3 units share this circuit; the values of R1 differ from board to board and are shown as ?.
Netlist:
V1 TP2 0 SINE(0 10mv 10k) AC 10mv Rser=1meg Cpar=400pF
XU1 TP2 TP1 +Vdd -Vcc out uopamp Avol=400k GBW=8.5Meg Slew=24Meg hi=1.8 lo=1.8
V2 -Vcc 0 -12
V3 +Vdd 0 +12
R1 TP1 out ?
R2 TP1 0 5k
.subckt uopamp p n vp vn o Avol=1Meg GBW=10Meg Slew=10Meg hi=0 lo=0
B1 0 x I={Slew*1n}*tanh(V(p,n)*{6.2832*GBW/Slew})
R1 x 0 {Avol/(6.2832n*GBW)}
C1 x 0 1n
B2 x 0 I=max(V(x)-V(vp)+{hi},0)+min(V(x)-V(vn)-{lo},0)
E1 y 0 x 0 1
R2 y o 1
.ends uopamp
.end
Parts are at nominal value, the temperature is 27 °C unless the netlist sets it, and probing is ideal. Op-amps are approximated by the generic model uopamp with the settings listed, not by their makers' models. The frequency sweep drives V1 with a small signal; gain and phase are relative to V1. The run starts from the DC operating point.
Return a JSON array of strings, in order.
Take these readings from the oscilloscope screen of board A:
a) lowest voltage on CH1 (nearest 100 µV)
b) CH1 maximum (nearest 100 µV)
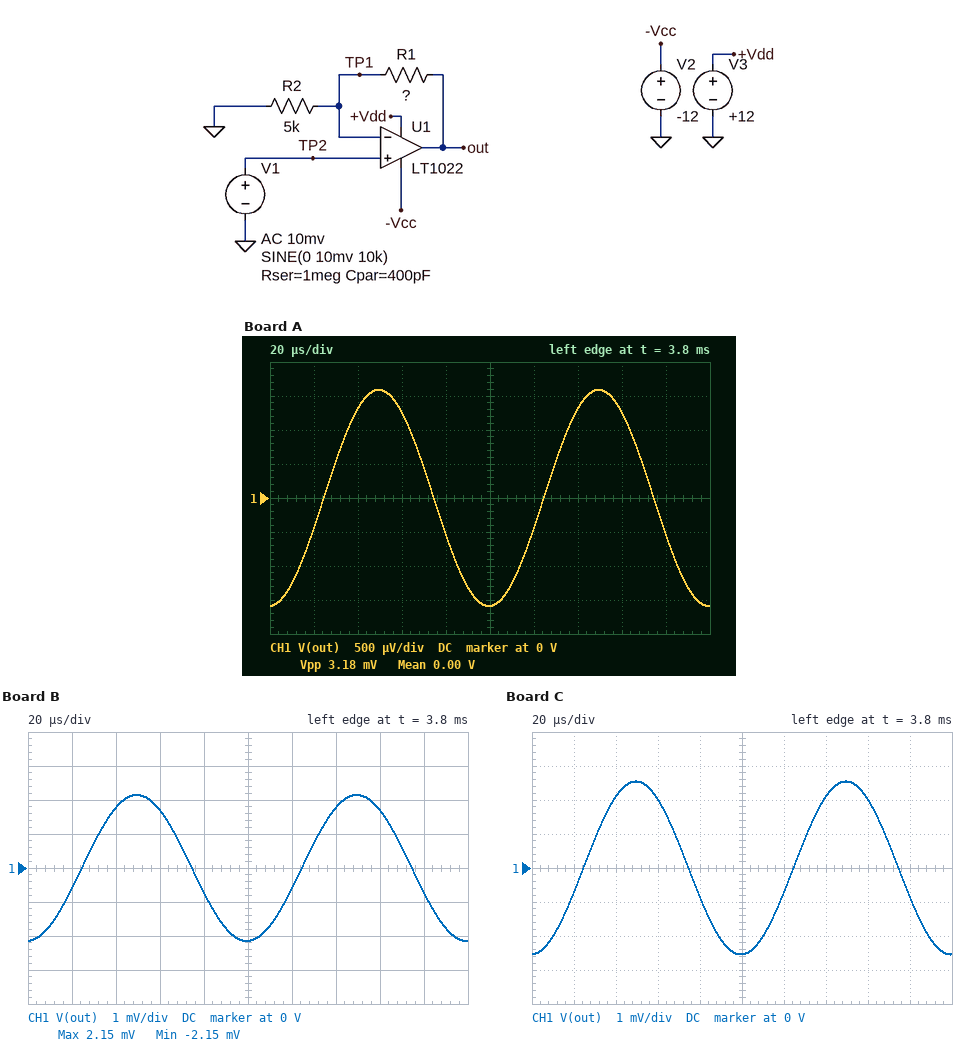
["-1.6 mV", "1.6 mV"]
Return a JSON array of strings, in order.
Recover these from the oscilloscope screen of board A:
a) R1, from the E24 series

["15 kΩ"]
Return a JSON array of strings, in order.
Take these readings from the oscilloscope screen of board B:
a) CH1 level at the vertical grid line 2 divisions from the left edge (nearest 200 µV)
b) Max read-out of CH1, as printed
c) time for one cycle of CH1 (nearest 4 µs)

["1.8 mV", "2.15 mV", "100 µs"]
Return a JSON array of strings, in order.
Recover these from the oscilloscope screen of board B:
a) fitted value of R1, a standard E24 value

["22 kΩ"]
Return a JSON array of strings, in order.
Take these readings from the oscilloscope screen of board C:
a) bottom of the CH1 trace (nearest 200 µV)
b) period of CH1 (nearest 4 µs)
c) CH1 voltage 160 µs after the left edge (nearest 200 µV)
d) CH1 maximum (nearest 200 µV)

["-2.6 mV", "100 µs", "2.0 mV", "2.6 mV"]
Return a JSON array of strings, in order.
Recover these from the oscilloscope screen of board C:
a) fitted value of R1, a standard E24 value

["27 kΩ"]
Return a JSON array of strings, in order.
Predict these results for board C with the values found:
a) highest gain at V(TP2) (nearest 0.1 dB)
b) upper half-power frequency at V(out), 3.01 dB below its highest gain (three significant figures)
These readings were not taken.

["0 dB", "398 Hz"]
